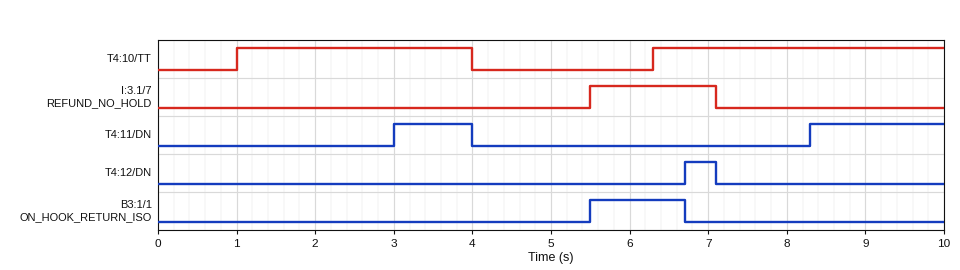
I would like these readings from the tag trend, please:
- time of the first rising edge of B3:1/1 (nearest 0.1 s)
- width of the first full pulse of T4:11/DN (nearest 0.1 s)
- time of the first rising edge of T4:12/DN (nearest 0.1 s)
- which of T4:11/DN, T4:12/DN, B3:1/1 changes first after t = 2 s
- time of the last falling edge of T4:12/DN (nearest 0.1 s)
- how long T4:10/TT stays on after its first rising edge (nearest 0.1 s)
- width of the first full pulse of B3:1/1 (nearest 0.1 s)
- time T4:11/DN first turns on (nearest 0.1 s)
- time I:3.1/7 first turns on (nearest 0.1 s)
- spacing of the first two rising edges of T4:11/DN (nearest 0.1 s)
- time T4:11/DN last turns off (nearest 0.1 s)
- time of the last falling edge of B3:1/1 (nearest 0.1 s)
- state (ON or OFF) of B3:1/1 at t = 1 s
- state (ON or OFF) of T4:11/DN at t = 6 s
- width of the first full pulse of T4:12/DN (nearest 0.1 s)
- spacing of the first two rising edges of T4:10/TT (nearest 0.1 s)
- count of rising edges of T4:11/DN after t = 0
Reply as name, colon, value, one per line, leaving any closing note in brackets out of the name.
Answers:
time of the first rising edge of B3:1/1: 5.5 s
width of the first full pulse of T4:11/DN: 1.0 s
time of the first rising edge of T4:12/DN: 6.7 s
which of T4:11/DN, T4:12/DN, B3:1/1 changes first after t = 2 s: T4:11/DN
time of the last falling edge of T4:12/DN: 7.1 s
how long T4:10/TT stays on after its first rising edge: 3.0 s
width of the first full pulse of B3:1/1: 1.2 s
time T4:11/DN first turns on: 3.0 s
time I:3.1/7 first turns on: 5.5 s
spacing of the first two rising edges of T4:11/DN: 5.3 s
time T4:11/DN last turns off: 4.0 s
time of the last falling edge of B3:1/1: 6.7 s
state (ON or OFF) of B3:1/1 at t = 1 s: OFF
state (ON or OFF) of T4:11/DN at t = 6 s: OFF
width of the first full pulse of T4:12/DN: 0.4 s
spacing of the first two rising edges of T4:10/TT: 5.3 s
count of rising edges of T4:11/DN after t = 0: 2
